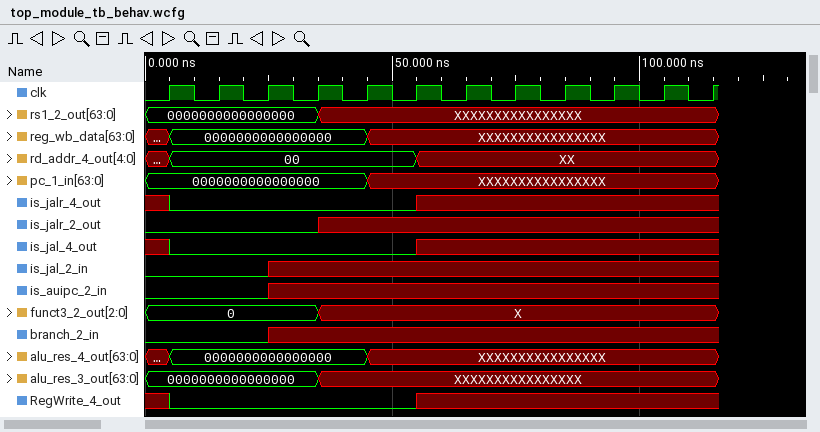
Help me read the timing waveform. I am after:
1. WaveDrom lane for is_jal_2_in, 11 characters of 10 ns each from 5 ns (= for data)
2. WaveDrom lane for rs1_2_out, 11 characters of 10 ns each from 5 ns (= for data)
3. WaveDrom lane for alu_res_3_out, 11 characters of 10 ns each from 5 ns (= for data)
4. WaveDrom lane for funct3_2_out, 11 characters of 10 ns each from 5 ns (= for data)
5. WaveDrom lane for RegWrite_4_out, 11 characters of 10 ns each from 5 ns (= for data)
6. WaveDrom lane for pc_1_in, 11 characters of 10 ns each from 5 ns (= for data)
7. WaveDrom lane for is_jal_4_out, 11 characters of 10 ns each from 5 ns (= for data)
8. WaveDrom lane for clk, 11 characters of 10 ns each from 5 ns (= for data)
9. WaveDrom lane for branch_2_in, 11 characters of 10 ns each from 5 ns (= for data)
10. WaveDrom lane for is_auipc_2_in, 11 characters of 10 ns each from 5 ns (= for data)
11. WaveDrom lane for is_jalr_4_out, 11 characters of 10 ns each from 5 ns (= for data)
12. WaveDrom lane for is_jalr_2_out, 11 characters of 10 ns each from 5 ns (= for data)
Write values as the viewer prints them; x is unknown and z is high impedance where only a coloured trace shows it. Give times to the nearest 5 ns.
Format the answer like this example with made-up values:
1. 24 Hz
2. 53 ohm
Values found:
1. {name: 'is_jal_2_in', wave: '0.x........'}
2. {name: 'rs1_2_out', wave: '=..x.......', data: '0000000000000000'}
3. {name: 'alu_res_3_out', wave: '=..x.......', data: '0000000000000000'}
4. {name: 'funct3_2_out', wave: '=..x.......', data: '0'}
5. {name: 'RegWrite_4_out', wave: '0....x.....'}
6. {name: 'pc_1_in', wave: '=...x......', data: '0000000000000000'}
7. {name: 'is_jal_4_out', wave: '0....x.....'}
8. {name: 'clk', wave: 'p..........'}
9. {name: 'branch_2_in', wave: '0.x........'}
10. {name: 'is_auipc_2_in', wave: '0.x........'}
11. {name: 'is_jalr_4_out', wave: '0....x.....'}
12. {name: 'is_jalr_2_out', wave: '0..x.......'}
